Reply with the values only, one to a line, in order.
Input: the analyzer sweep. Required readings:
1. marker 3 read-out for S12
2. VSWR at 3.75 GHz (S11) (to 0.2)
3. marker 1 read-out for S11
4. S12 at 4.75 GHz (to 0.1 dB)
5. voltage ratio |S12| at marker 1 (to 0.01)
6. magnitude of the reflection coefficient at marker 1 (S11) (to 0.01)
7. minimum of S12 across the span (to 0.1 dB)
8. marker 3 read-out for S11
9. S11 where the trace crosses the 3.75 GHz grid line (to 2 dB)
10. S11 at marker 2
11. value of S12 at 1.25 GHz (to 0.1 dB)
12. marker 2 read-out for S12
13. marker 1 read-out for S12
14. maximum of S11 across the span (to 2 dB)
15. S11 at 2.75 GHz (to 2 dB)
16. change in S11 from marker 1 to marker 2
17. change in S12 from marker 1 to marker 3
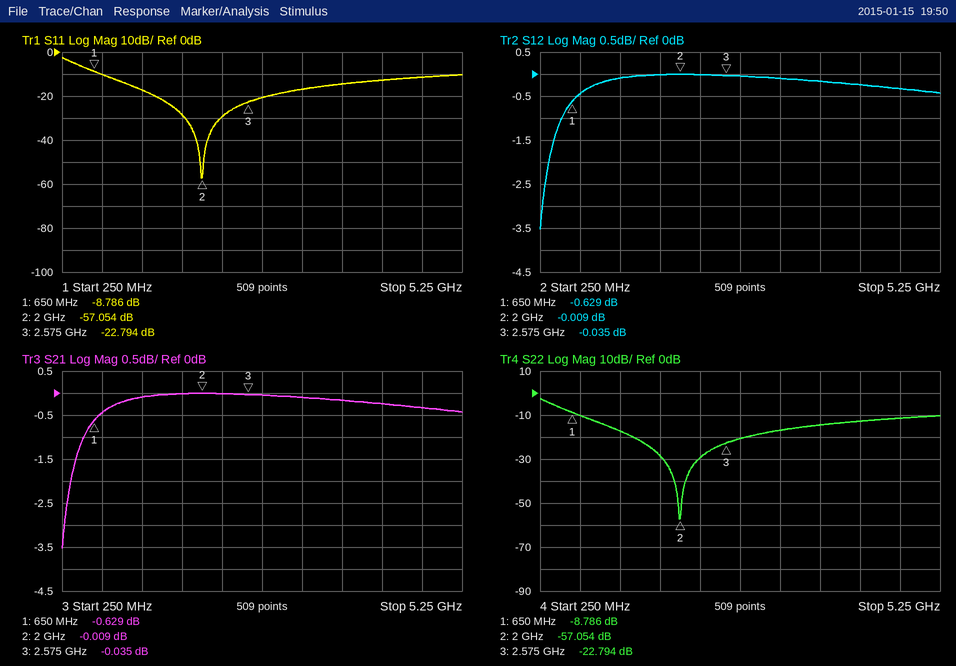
-0.035 dB
1.4
-8.786 dB
-0.3 dB
0.93
0.36
-3.5 dB
-22.794 dB
-14 dB
-57.054 dB
-0.1 dB
-0.009 dB
-0.629 dB
-2 dB
-20 dB
-48.268 dB
0.594 dB
